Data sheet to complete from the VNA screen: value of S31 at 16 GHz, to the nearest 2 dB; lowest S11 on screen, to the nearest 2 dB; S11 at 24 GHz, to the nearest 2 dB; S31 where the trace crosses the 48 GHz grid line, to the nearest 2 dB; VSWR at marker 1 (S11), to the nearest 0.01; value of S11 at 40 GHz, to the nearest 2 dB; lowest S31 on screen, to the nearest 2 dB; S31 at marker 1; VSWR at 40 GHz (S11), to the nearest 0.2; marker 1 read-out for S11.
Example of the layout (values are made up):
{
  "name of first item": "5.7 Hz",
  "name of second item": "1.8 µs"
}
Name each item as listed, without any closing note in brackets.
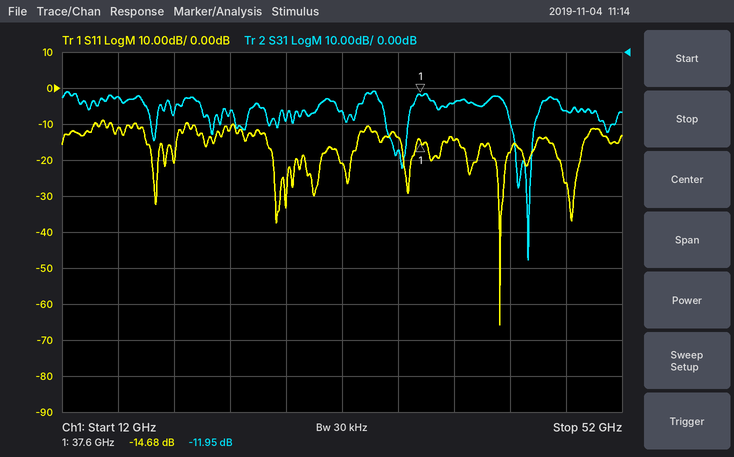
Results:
{
  "value of S31 at 16 GHz, to the nearest 2 dB": "-12 dB",
  "lowest S11 on screen, to the nearest 2 dB": "-66 dB",
  "S11 at 24 GHz, to the nearest 2 dB": "-12 dB",
  "S31 where the trace crosses the 48 GHz grid line, to the nearest 2 dB": "-16 dB",
  "VSWR at marker 1 (S11), to the nearest 0.01": "1.45",
  "value of S11 at 40 GHz, to the nearest 2 dB": "-14 dB",
  "lowest S31 on screen, to the nearest 2 dB": "-58 dB",
  "S31 at marker 1": "-11.95 dB",
  "VSWR at 40 GHz (S11), to the nearest 0.2": "1.4",
  "marker 1 read-out for S11": "-14.68 dB"
}
